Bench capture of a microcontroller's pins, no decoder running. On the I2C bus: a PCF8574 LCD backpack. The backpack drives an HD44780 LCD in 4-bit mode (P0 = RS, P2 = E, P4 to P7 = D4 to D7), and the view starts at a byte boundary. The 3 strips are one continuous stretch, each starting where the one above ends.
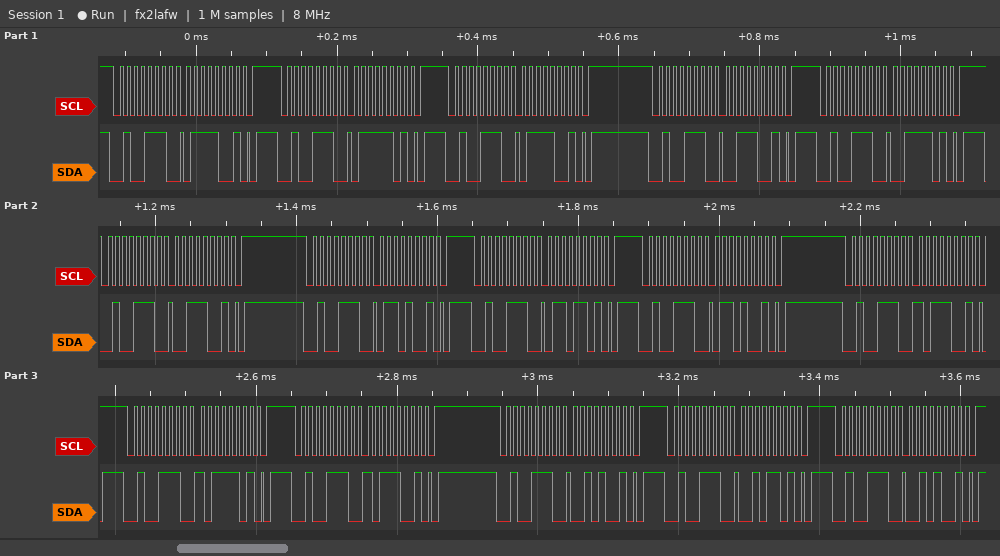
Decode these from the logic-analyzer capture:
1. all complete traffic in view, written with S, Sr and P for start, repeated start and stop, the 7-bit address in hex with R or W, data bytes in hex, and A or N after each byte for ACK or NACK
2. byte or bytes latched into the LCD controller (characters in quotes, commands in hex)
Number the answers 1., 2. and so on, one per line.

1. S 27W A 79 A P S 27W A 7D A P S 27W A 79 A P S 27W A 39 A P S 27W A 3D A P S 27W A 39 A P S 27W A 69 A P S 27W A 6D A P S 27W A 69 A P S 27W A B9 A P S 27W A BD A P S 27W A B9 A P S 27W A 29 A P S 27W A 2D A P S 27W A 29 A P
2. 's' 'k'
